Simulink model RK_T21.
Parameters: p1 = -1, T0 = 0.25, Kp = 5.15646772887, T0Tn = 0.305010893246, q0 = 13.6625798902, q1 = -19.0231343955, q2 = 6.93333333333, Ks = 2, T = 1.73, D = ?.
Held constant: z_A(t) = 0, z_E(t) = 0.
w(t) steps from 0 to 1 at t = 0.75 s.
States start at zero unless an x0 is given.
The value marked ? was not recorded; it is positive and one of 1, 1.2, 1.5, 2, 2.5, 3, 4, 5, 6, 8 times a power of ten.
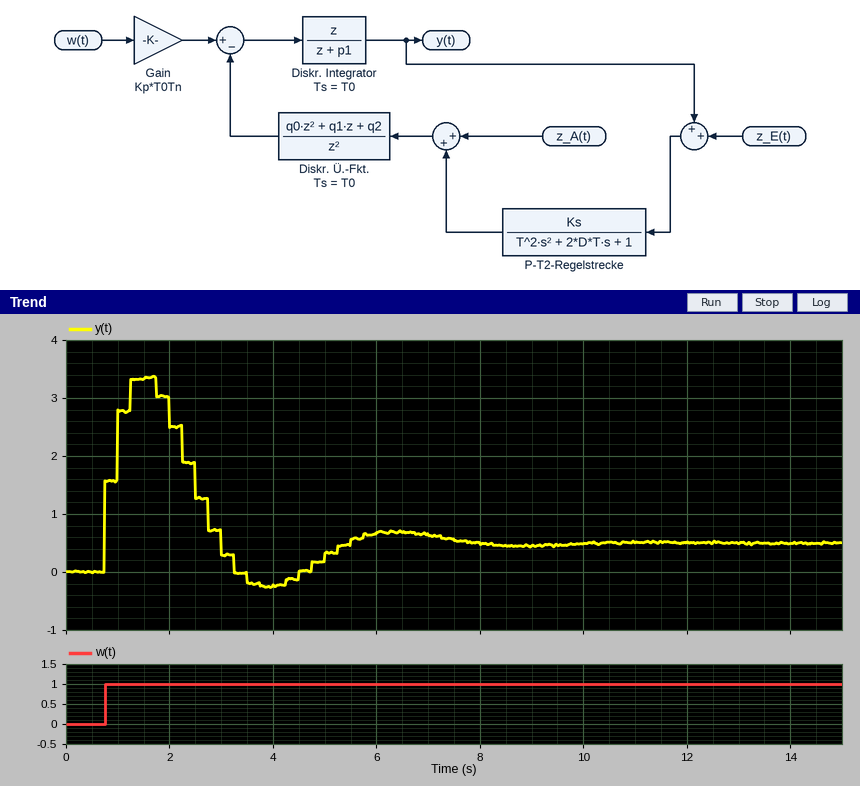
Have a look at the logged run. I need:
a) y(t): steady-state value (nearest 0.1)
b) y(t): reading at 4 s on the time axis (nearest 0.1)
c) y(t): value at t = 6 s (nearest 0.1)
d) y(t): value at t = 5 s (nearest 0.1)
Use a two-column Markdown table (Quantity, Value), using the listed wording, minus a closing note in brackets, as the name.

| Quantity | Value |
|---|---|
| y(t): steady-state value | 0.5 |
| y(t): reading at 4 s on the time axis | -0.2 |
| y(t): value at t = 6 s | 0.7 |
| y(t): value at t = 5 s | 0.3 |
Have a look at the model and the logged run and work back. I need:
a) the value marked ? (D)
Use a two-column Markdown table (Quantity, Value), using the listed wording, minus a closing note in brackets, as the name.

| Quantity | Value |
|---|---|
| the value marked ? | 2 |
